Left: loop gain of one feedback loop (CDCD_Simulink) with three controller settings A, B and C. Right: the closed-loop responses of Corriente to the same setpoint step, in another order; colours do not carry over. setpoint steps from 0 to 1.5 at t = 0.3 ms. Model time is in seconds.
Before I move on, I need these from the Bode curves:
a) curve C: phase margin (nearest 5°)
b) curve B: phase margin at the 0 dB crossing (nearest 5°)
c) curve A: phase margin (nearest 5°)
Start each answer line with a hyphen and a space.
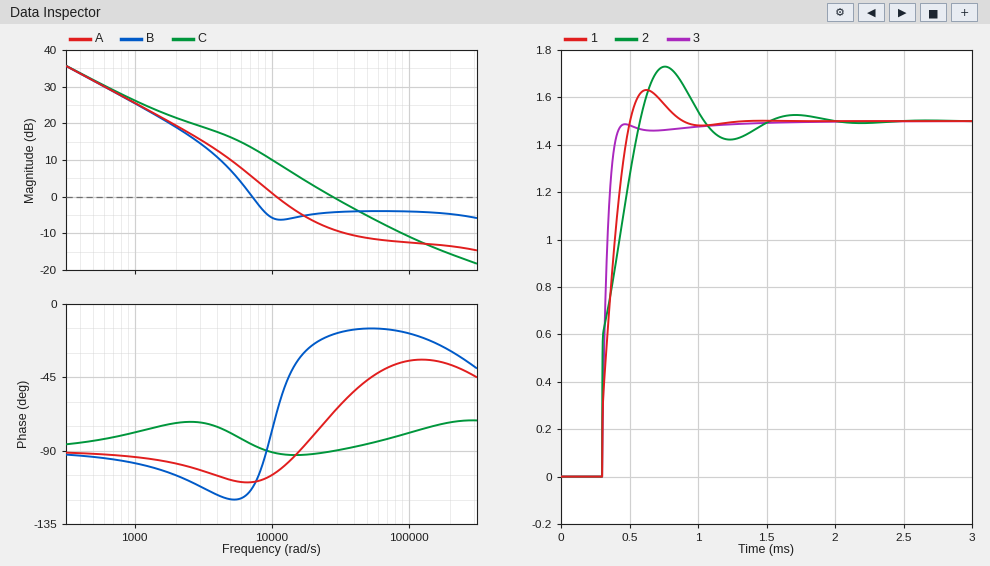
- 90°
- 65°
- 75°
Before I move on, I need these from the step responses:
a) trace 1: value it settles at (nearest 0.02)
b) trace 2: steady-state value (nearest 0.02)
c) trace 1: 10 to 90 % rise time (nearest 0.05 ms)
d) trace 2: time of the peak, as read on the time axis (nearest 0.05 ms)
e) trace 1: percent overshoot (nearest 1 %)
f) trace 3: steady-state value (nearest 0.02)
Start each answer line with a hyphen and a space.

- 1.50
- 1.50
- 0.15 ms
- 0.75 ms
- 9 %
- 1.50
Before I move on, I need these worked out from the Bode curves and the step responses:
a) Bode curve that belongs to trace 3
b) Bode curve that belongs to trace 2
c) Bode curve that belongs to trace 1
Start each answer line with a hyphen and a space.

- C
- B
- A
